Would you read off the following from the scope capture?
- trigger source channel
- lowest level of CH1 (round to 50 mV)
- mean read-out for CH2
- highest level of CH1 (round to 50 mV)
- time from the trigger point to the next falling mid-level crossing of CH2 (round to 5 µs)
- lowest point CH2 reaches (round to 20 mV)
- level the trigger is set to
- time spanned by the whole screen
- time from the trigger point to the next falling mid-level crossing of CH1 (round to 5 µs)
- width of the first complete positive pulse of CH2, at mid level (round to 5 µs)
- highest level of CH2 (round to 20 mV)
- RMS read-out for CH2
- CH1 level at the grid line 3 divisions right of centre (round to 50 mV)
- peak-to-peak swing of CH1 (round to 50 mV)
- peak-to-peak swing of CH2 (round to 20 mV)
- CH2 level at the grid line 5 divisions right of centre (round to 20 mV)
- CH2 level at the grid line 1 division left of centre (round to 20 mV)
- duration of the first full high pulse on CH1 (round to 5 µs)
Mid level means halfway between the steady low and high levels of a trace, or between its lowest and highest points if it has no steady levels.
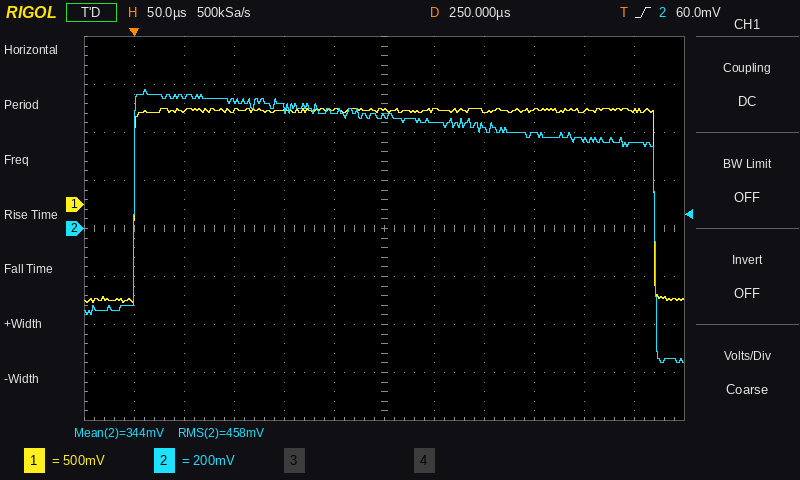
CH2
-1.00 V
344 mV
1.00 V
520 µs
-560 mV
60.0 mV
600 µs
520 µs
520 µs
580 mV
458 mV
1.00 V
2.00 V
1.14 V
360 mV
480 mV
520 µs
